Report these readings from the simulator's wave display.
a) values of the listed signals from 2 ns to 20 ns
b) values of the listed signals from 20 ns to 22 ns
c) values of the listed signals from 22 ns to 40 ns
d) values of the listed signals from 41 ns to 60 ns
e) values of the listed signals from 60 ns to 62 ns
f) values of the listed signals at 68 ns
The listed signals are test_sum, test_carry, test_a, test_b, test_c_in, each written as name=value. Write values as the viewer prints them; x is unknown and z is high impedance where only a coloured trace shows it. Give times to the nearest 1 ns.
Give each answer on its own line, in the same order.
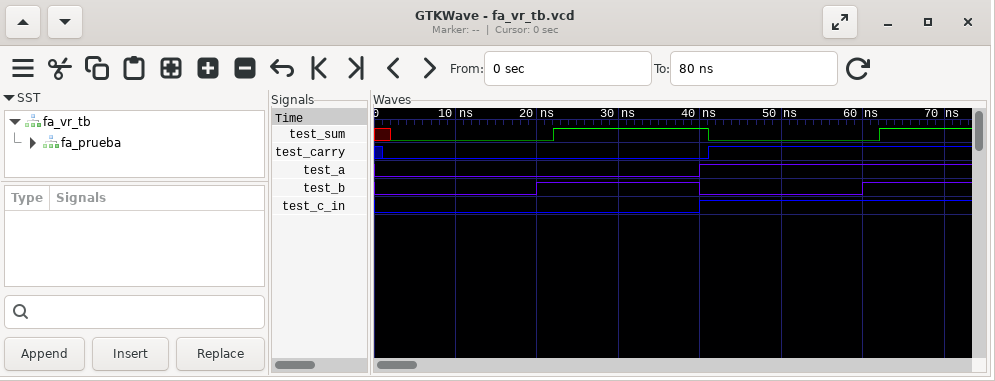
test_sum=0, test_carry=0, test_a=0, test_b=0, test_c_in=0
test_sum=0, test_carry=0, test_a=0, test_b=1, test_c_in=0
test_sum=1, test_carry=0, test_a=0, test_b=1, test_c_in=0
test_sum=0, test_carry=1, test_a=1, test_b=0, test_c_in=1
test_sum=0, test_carry=1, test_a=1, test_b=1, test_c_in=1
test_sum=1, test_carry=1, test_a=1, test_b=1, test_c_in=1
